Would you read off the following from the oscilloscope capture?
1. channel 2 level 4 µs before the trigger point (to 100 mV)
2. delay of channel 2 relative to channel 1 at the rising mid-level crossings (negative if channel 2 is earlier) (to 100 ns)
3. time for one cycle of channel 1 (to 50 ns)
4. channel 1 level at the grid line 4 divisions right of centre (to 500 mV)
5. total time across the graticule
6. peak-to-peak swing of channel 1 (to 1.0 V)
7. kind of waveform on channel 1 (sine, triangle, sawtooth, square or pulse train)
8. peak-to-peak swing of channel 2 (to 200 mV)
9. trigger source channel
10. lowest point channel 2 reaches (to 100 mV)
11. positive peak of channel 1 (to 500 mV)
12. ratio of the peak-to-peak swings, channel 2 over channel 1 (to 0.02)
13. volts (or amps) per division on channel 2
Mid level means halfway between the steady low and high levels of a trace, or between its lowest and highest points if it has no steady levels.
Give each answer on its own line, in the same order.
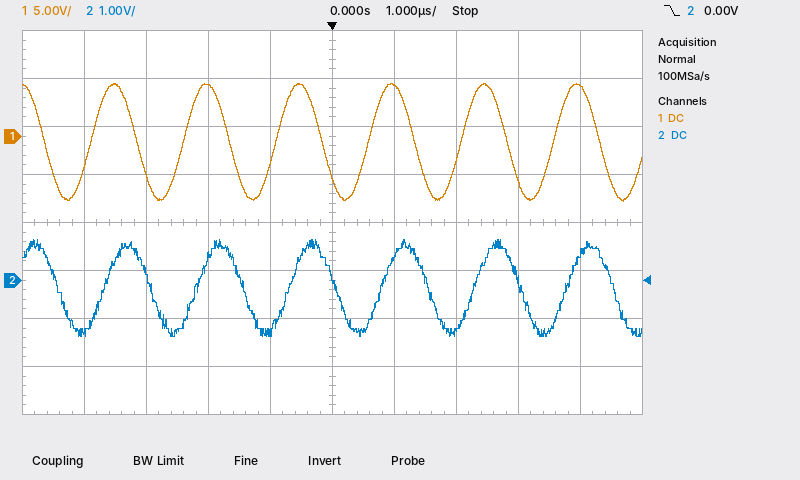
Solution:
-1.1 V
+200 ns
1.50 µs
5.0 V
10 µs
12.0 V
sine
2.0 V
channel 2
-1.2 V
5.5 V
0.16
1 V
